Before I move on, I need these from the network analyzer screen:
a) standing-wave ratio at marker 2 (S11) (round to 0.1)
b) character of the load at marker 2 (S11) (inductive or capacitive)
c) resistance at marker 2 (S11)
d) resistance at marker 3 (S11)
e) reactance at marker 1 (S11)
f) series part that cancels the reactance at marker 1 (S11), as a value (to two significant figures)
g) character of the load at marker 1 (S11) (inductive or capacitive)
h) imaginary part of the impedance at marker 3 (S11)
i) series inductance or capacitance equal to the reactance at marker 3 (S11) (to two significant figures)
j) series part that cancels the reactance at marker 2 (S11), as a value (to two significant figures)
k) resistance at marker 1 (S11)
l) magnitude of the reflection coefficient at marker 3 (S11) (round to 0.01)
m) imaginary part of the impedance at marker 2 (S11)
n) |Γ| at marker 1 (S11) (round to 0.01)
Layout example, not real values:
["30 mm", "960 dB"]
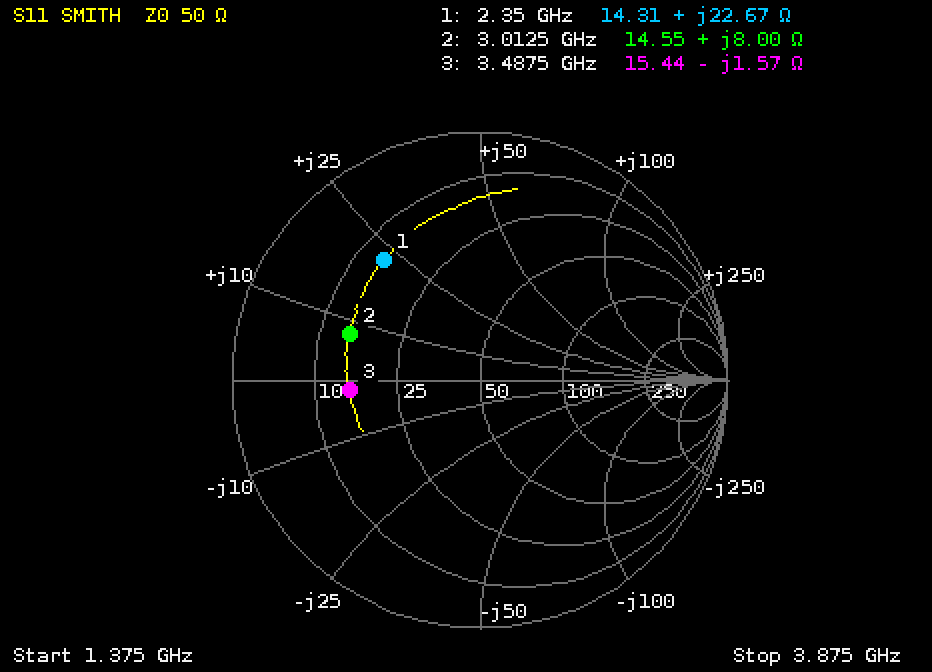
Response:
["3.5", "inductive", "14.55 Ω", "15.44 Ω", "+22.67 Ω", "3.0 pF", "inductive", "-1.57 Ω", "29 pF", "6.6 pF", "14.31 Ω", "0.53", "+8.00 Ω", "0.62"]
